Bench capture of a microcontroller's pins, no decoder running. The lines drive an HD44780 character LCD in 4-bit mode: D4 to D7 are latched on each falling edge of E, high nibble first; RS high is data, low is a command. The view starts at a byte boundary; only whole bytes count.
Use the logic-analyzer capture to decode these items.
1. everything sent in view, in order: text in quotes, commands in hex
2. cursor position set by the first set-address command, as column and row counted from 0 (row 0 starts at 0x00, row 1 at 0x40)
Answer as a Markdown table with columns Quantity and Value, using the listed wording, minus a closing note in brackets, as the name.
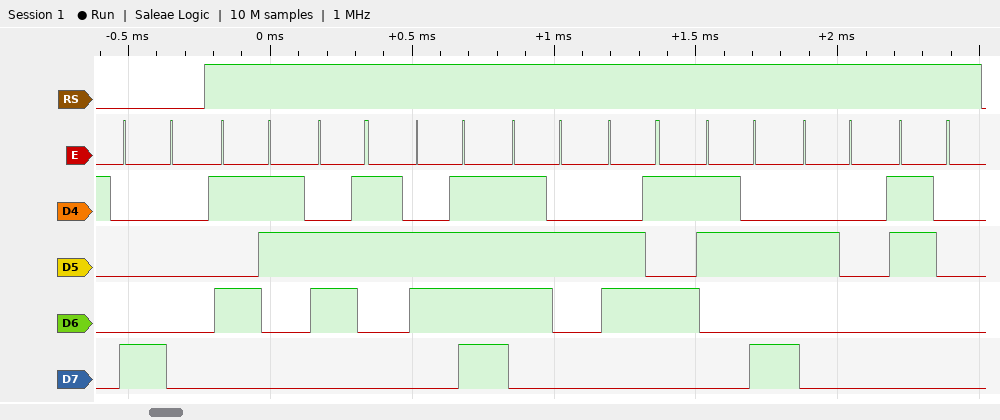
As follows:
| Quantity | Value |
|---|---|
| everything sent in view, in order: text in quotes, commands in hex | 0x80 "Score: 0" |
| cursor position set by the first set-address command, as column and row counted from 0 | column 0, row 0 |
